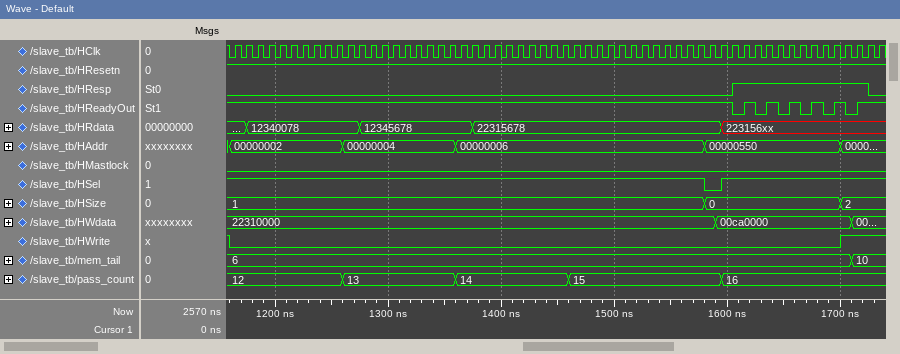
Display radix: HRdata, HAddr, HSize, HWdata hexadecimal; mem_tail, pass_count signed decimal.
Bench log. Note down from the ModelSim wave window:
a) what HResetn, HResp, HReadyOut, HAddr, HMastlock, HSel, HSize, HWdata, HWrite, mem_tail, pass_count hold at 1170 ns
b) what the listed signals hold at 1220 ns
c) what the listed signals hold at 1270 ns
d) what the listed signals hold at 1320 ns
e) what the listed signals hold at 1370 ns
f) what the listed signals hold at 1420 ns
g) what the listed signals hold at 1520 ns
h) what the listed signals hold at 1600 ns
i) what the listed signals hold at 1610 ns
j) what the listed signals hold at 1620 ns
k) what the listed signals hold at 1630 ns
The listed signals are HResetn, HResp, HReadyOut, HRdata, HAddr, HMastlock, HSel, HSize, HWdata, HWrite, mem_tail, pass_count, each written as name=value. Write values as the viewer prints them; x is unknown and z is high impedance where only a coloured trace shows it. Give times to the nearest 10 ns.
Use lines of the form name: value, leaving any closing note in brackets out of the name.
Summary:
what HResetn, HResp, HReadyOut, HAddr, HMastlock, HSel, HSize, HWdata, HWrite, mem_tail, pass_count hold at 1170 ns: HResetn=1, HResp=0, HReadyOut=1, HAddr=00000002, HMastlock=0, HSel=1, HSize=1, HWdata=22310000, HWrite=0, mem_tail=6, pass_count=12
what the listed signals hold at 1220 ns: HResetn=1, HResp=0, HReadyOut=1, HRdata=12340078, HAddr=00000002, HMastlock=0, HSel=1, HSize=1, HWdata=22310000, HWrite=0, mem_tail=6, pass_count=12
what the listed signals hold at 1270 ns: HResetn=1, HResp=0, HReadyOut=1, HRdata=12340078, HAddr=00000004, HMastlock=0, HSel=1, HSize=1, HWdata=22310000, HWrite=0, mem_tail=6, pass_count=13
what the listed signals hold at 1320 ns: HResetn=1, HResp=0, HReadyOut=1, HRdata=12345678, HAddr=00000004, HMastlock=0, HSel=1, HSize=1, HWdata=22310000, HWrite=0, mem_tail=6, pass_count=13
what the listed signals hold at 1370 ns: HResetn=1, HResp=0, HReadyOut=1, HRdata=12345678, HAddr=00000006, HMastlock=0, HSel=1, HSize=1, HWdata=22310000, HWrite=0, mem_tail=6, pass_count=14
what the listed signals hold at 1420 ns: HResetn=1, HResp=0, HReadyOut=1, HRdata=22315678, HAddr=00000006, HMastlock=0, HSel=1, HSize=1, HWdata=22310000, HWrite=0, mem_tail=6, pass_count=14
what the listed signals hold at 1520 ns: HResetn=1, HResp=0, HReadyOut=1, HRdata=22315678, HAddr=00000006, HMastlock=0, HSel=1, HSize=1, HWdata=22310000, HWrite=0, mem_tail=6, pass_count=15
what the listed signals hold at 1600 ns: HResetn=1, HResp=0, HReadyOut=1, HRdata=223156xx, HAddr=00000550, HMastlock=0, HSel=1, HSize=0, HWdata=00ca0000, HWrite=0, mem_tail=6, pass_count=16
what the listed signals hold at 1610 ns: HResetn=1, HResp=1, HReadyOut=0, HRdata=223156xx, HAddr=00000550, HMastlock=0, HSel=1, HSize=0, HWdata=00ca0000, HWrite=0, mem_tail=6, pass_count=16
what the listed signals hold at 1620 ns: HResetn=1, HResp=1, HReadyOut=1, HRdata=223156xx, HAddr=00000550, HMastlock=0, HSel=1, HSize=0, HWdata=00ca0000, HWrite=0, mem_tail=6, pass_count=16
what the listed signals hold at 1630 ns: HResetn=1, HResp=1, HReadyOut=0, HRdata=223156xx, HAddr=00000550, HMastlock=0, HSel=1, HSize=0, HWdata=00ca0000, HWrite=0, mem_tail=6, pass_count=16
